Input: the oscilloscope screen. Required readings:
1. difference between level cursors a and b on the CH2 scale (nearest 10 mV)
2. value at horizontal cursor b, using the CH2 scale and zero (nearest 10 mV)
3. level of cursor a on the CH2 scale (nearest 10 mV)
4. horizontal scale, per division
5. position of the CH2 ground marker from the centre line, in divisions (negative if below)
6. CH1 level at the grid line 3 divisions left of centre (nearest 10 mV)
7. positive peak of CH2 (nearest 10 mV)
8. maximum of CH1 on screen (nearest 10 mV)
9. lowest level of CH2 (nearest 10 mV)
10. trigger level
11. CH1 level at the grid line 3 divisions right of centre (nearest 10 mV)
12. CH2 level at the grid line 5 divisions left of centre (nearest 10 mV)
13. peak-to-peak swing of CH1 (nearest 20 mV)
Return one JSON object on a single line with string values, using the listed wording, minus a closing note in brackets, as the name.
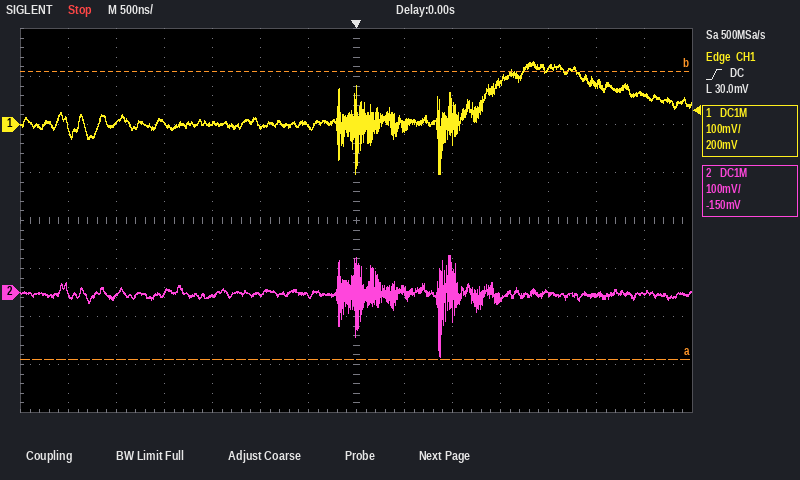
{"difference between level cursors a and b on the CH2 scale": "600 mV", "value at horizontal cursor b, using the CH2 scale and zero": "460 mV", "level of cursor a on the CH2 scale": "-140 mV", "horizontal scale, per division": "500 ns", "position of the CH2 ground marker from the centre line, in divisions": "-1.5 div", "CH1 level at the grid line 3 divisions left of centre": "0 mV", "positive peak of CH2": "80 mV", "maximum of CH1 on screen": "130 mV", "lowest level of CH2": "-140 mV", "trigger level": "30.0 mV", "CH1 level at the grid line 3 divisions right of centre": "90 mV", "CH2 level at the grid line 5 divisions left of centre": "-10 mV", "peak-to-peak swing of CH1": "240 mV"}
